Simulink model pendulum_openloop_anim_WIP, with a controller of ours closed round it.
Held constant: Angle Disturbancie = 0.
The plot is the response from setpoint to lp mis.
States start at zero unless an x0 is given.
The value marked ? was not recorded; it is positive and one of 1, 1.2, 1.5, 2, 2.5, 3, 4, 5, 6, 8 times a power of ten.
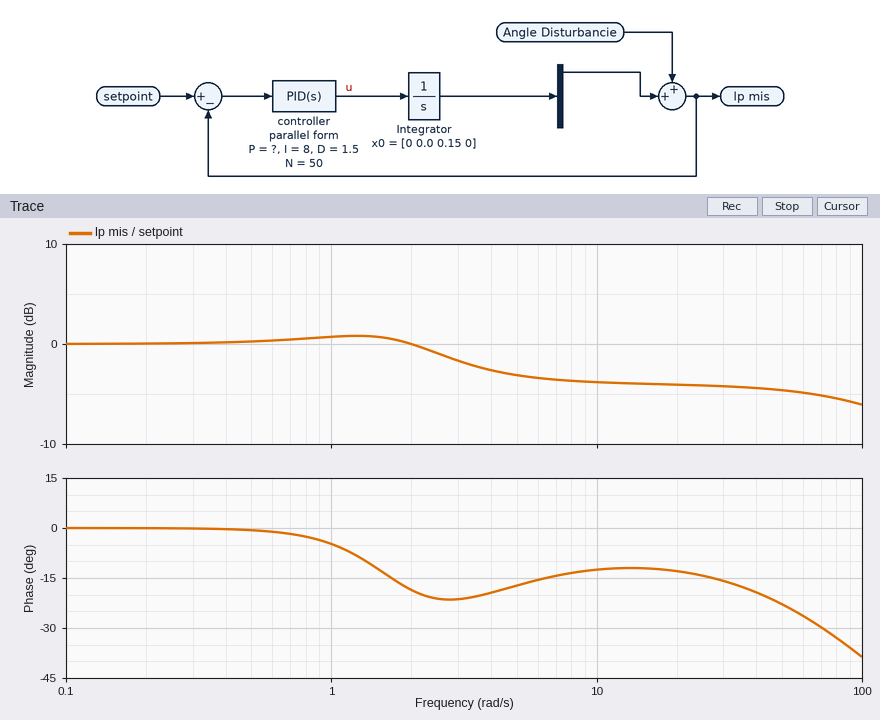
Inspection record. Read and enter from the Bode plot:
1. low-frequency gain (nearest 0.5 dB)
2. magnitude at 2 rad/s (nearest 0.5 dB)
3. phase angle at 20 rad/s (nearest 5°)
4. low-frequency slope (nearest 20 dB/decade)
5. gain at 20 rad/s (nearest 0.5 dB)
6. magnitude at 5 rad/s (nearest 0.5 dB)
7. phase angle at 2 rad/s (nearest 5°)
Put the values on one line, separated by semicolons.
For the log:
0.0 dB; 0.0 dB; -15°; 0 dB/decade; -4.0 dB; -3.0 dB; -20°
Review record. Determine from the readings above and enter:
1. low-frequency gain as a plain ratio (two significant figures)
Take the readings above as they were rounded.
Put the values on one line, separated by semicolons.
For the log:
1.0
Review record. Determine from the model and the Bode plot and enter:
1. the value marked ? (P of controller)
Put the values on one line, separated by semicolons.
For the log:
6
